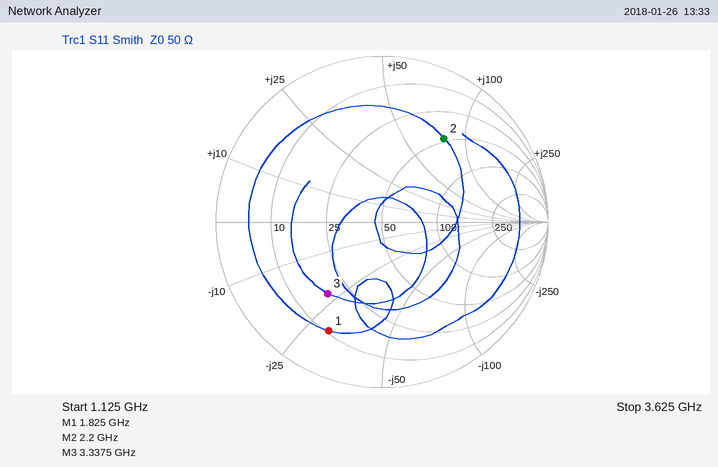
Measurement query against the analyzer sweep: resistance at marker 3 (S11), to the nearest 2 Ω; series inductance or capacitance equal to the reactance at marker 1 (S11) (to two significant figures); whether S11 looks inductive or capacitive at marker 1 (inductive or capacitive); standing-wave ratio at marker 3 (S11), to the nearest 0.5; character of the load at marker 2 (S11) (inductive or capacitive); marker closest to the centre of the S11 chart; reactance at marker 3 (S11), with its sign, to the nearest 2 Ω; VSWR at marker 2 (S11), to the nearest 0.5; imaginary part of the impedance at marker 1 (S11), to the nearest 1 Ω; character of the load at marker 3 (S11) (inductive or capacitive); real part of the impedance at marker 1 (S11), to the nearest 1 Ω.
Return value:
18 Ω
2.9 pF
capacitive
3.5
inductive
marker 3
-22 Ω
4.5
-30 Ω
capacitive
11 Ω
